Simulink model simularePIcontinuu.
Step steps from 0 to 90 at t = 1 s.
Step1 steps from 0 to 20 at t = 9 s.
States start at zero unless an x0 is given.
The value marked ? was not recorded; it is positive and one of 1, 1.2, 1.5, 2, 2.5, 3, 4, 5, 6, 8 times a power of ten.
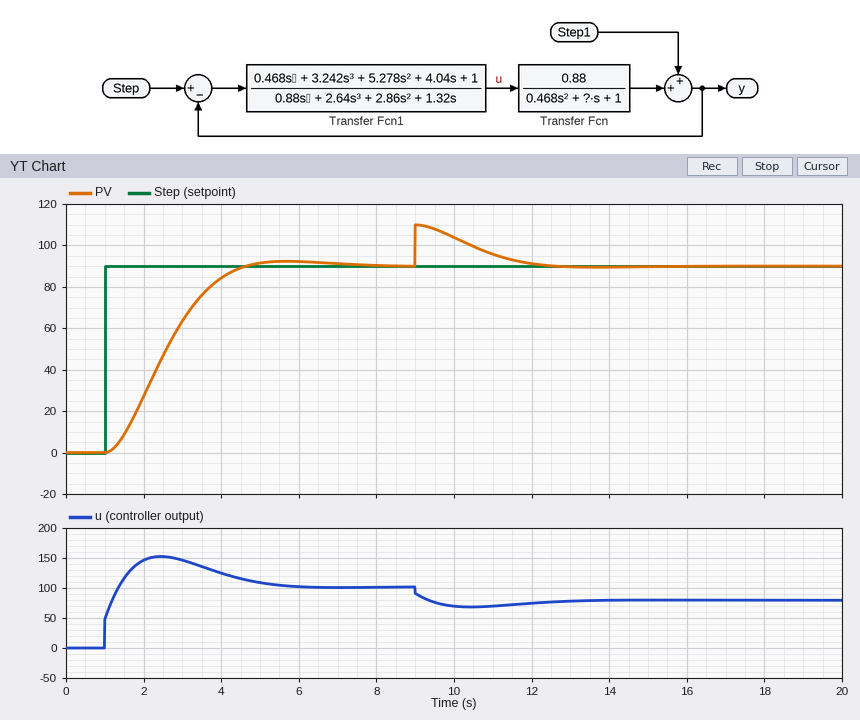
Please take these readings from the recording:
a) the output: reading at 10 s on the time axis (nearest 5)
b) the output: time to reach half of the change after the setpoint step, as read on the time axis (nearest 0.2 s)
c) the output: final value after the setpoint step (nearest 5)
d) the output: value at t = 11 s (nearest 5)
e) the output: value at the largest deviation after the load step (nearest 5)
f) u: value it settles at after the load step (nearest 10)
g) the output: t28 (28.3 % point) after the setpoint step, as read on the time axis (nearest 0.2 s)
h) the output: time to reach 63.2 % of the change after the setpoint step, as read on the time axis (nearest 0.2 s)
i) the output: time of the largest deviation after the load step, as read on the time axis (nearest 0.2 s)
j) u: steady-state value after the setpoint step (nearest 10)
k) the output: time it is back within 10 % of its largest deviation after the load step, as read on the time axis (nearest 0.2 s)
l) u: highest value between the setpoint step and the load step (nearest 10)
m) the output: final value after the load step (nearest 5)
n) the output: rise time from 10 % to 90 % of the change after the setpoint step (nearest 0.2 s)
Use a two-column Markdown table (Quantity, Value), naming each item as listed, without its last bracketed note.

| Quantity | Value |
|---|---|
| the output: reading at 10 s on the time axis | 105 |
| the output: time to reach half of the change after the setpoint step, as read on the time axis | 2.4 s |
| the output: final value after the setpoint step | 90 |
| the output: value at t = 11 s | 95 |
| the output: value at the largest deviation after the load step | 110 |
| u: value it settles at after the load step | 80 |
| the output: t28 (28.3 % point) after the setpoint step, as read on the time axis | 2.0 s |
| the output: time to reach 63.2 % of the change after the setpoint step, as read on the time axis | 2.8 s |
| the output: time of the largest deviation after the load step, as read on the time axis | 9.0 s |
| u: steady-state value after the setpoint step | 100 |
| the output: time it is back within 10 % of its largest deviation after the load step, as read on the time axis | 11.8 s |
| u: highest value between the setpoint step and the load step | 150 |
| the output: final value after the load step | 90 |
| the output: rise time from 10 % to 90 % of the change after the setpoint step | 2.2 s |
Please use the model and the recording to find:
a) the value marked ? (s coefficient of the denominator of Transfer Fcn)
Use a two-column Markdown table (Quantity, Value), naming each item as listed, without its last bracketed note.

| Quantity | Value |
|---|---|
| the value marked ? | 2.5 |
